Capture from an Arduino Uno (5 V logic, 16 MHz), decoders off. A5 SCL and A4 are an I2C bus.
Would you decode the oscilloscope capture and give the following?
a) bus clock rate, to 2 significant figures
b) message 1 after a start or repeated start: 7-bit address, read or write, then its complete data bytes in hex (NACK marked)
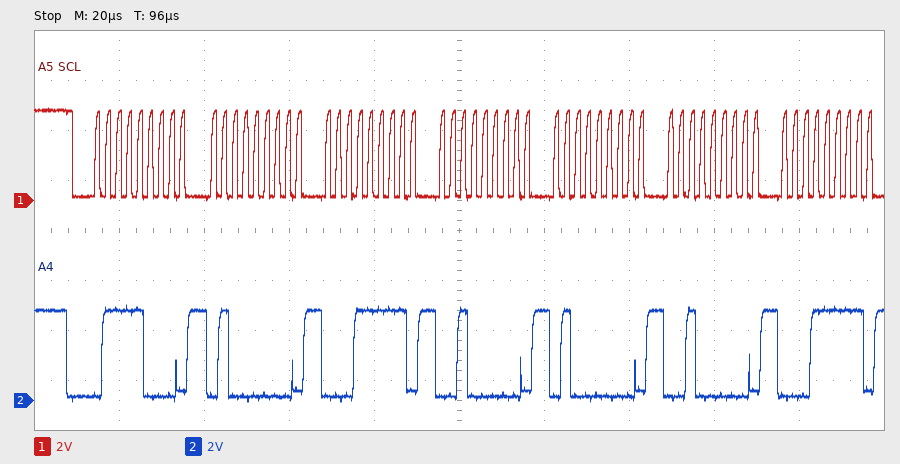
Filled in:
400 kHz
0x3C write: 40 1F 20 40 20 1F
